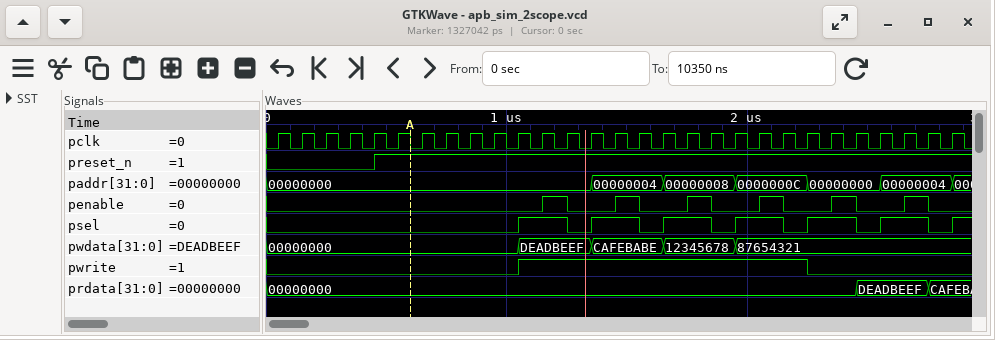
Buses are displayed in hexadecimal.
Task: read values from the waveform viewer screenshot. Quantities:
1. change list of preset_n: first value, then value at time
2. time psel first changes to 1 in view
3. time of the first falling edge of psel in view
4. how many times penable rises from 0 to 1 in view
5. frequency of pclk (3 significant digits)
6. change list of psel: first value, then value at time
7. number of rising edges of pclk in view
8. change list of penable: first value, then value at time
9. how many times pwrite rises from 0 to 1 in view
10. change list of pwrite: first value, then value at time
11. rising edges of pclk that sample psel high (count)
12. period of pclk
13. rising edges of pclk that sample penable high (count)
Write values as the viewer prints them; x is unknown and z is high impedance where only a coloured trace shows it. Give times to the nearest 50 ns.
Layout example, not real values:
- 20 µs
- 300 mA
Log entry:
- 0, 1 at 450 ns
- 1050 ns
- 1250 ns
- 6
- 10.0 MHz
- 0, 1 at 1050 ns, 0 at 1250 ns, 1 at 1350 ns, 0 at 1550 ns, 1 at 1650 ns, 0 at 1850 ns, 1 at 1950 ns, 0 at 2150 ns, 1 at 2250 ns, 0 at 2450 ns, 1 at 2550 ns, 0 at 2750 ns, 1 at 2850 ns
- 29
- 0, 1 at 1150 ns, 0 at 1250 ns, 1 at 1450 ns, 0 at 1550 ns, 1 at 1750 ns, 0 at 1850 ns, 1 at 2050 ns, 0 at 2150 ns, 1 at 2350 ns, 0 at 2450 ns, 1 at 2650 ns, 0 at 2750 ns
- 1
- 0, 1 at 1050 ns, 0 at 2250 ns
- 12
- 100 ns
- 6
